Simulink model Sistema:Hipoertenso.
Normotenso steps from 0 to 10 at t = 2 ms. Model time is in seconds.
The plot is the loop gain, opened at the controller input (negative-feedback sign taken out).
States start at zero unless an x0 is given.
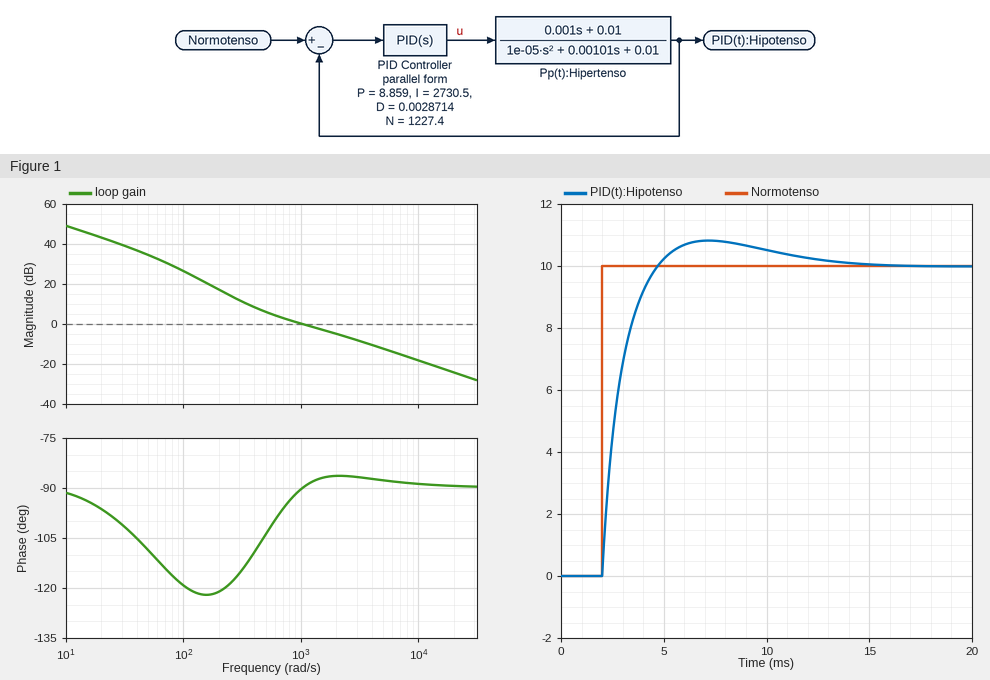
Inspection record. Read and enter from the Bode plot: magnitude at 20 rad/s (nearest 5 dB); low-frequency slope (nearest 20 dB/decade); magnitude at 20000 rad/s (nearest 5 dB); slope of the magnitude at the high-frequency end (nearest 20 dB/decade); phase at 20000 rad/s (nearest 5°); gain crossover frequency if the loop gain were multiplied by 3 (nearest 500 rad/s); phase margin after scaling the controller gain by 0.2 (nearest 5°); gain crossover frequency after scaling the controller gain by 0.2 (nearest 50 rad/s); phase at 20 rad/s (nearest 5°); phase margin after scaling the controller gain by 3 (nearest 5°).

45 dB
-20 dB/decade
-25 dB
-20 dB/decade
-90°
3500 rad/s
60°
250 rad/s
-95°
95°
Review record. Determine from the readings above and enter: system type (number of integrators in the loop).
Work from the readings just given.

1
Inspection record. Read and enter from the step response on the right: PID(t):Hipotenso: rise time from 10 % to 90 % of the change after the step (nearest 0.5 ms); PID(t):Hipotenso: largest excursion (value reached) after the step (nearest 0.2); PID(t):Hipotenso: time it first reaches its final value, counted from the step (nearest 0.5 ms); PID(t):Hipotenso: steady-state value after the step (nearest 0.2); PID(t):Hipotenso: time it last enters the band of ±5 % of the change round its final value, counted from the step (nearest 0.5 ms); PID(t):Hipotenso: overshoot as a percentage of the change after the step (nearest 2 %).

2.0 ms
10.8
2.5 ms
10.0
8.0 ms
8 %
